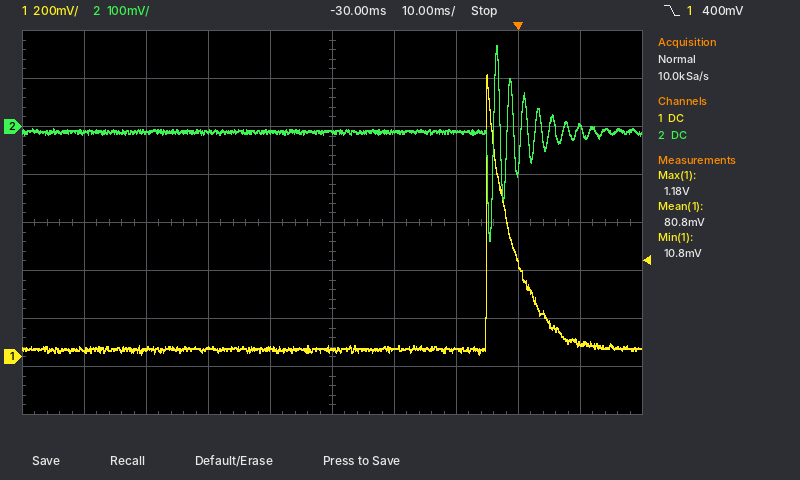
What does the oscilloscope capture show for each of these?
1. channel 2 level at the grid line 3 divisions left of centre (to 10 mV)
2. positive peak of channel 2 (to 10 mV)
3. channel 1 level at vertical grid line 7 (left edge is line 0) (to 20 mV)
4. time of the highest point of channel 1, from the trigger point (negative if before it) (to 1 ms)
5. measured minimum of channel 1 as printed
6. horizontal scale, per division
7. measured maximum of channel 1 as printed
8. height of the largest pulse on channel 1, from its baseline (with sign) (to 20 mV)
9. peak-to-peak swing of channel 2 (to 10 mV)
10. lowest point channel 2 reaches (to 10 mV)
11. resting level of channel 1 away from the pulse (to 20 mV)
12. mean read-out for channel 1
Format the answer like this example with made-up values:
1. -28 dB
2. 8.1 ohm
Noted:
1. -10 mV
2. 170 mV
3. 40 mV
4. -5 ms
5. 10.8 mV
6. 10 ms
7. 1.18 V
8. +1.14 V
9. 410 mV
10. -240 mV
11. 40 mV
12. 80.8 mV
